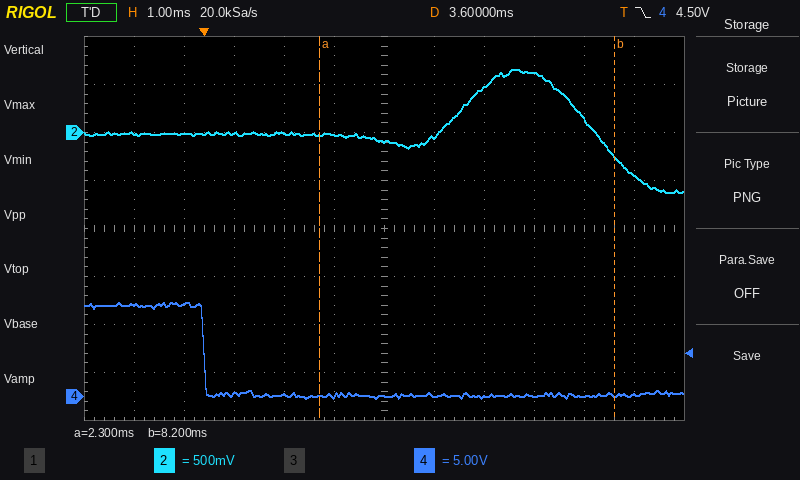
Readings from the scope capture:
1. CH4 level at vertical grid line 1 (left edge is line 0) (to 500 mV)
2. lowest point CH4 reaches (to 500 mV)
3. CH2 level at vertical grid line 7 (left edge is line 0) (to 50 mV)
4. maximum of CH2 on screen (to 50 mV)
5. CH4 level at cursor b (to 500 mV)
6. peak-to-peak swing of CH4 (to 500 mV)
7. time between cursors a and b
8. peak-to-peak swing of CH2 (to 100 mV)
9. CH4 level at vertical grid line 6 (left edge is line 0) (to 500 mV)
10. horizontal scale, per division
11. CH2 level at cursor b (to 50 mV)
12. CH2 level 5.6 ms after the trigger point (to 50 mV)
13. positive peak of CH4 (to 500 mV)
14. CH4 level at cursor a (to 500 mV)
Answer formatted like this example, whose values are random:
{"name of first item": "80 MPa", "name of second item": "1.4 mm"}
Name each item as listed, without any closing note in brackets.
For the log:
{"CH4 level at vertical grid line 1 (left edge is line 0)": "9.5 V", "lowest point CH4 reaches": "0.0 V", "CH2 level at vertical grid line 7 (left edge is line 0)": "-50 mV", "maximum of CH2 on screen": "650 mV", "CH4 level at cursor b": "0.0 V", "peak-to-peak swing of CH4": "10.0 V", "time between cursors a and b": "5.9 ms", "peak-to-peak swing of CH2": "1.30 V", "CH4 level at vertical grid line 6 (left edge is line 0)": "0.0 V", "horizontal scale, per division": "1 ms", "CH2 level at cursor b": "-250 mV", "CH2 level 5.6 ms after the trigger point": "450 mV", "positive peak of CH4": "10.0 V", "CH4 level at cursor a": "0.0 V"}
